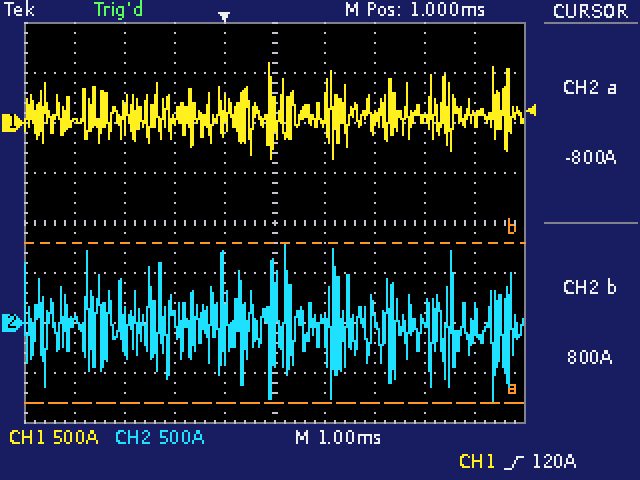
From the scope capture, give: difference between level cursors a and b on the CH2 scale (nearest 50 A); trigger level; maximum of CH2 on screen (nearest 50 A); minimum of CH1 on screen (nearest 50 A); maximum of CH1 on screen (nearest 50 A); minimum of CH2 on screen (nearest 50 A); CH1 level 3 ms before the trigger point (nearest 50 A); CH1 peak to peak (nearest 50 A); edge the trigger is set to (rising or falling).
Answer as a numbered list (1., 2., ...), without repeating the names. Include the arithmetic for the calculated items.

1. 1.60 kA
2. 120 A
3. 800 A
4. -350 A
5. 600 A
6. -800 A
7. 0 A
8. 600 A − (-350 A) = 950 A
9. rising
